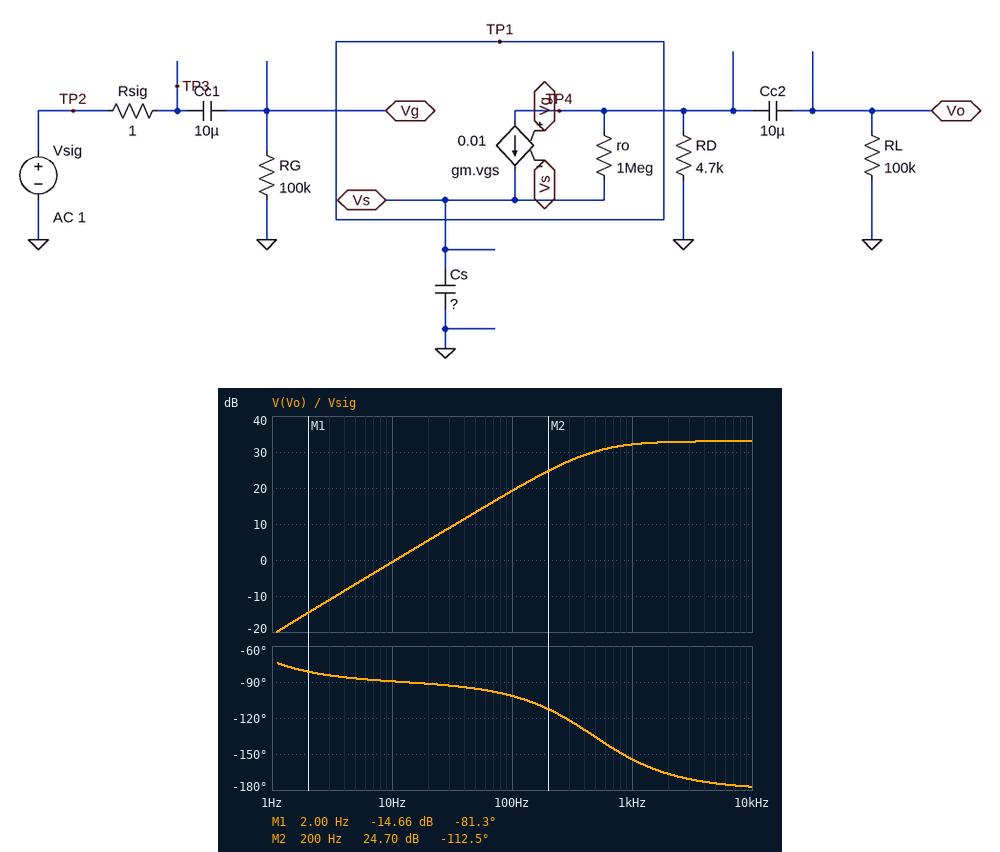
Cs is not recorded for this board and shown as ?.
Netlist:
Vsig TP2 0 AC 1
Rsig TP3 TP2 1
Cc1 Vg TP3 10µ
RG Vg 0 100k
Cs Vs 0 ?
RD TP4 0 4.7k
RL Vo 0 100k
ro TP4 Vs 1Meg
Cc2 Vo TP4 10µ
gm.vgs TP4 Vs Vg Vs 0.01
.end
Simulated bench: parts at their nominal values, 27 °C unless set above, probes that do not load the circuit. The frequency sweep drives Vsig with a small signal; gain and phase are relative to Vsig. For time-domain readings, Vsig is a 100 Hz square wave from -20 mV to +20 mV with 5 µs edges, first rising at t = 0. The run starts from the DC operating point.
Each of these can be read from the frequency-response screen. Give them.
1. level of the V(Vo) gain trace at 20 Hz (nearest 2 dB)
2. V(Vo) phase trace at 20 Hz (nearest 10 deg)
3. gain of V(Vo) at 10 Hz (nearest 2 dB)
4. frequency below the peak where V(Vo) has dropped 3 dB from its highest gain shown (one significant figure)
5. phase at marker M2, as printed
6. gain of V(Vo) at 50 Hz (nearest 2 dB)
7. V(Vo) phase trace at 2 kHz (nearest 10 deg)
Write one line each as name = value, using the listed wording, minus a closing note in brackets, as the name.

level of the V(Vo) gain trace at 20 Hz = 6 dB
V(Vo) phase trace at 20 Hz = -90 deg
gain of V(Vo) at 10 Hz = 0 dB
frequency below the peak where V(Vo) has dropped 3 dB from its highest gain shown = 500 Hz
phase at marker M2, as printed = -112.5 deg
gain of V(Vo) at 50 Hz = 14 dB
V(Vo) phase trace at 2 kHz = -170 deg
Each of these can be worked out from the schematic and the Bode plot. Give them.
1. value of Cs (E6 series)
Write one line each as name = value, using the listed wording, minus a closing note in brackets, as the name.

value of Cs = 3.3 µF
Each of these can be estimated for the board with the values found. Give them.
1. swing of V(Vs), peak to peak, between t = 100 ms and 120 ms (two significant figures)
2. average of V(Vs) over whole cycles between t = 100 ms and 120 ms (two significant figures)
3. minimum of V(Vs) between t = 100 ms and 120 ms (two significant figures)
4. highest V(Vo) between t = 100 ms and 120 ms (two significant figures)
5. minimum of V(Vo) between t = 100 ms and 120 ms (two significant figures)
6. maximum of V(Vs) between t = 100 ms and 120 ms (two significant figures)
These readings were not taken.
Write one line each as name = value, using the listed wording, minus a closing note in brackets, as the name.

swing of V(Vs), peak to peak, between t = 100 ms and 120 ms = 40 mV
average of V(Vs) over whole cycles between t = 100 ms and 120 ms = 18 mV
minimum of V(Vs) between t = 100 ms and 120 ms = -2.3 mV
highest V(Vo) between t = 100 ms and 120 ms = 1.8 V
minimum of V(Vo) between t = 100 ms and 120 ms = -1.8 V
maximum of V(Vs) between t = 100 ms and 120 ms = 38 mV
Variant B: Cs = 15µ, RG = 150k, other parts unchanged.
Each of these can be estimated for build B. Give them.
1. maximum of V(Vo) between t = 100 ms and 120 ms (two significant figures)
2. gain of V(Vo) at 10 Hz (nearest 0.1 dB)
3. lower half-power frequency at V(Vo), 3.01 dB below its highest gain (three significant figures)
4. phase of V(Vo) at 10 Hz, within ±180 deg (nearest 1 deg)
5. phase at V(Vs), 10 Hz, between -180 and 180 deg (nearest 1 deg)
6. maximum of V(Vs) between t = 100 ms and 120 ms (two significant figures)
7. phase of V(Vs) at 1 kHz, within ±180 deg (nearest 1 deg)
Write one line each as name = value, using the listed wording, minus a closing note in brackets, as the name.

maximum of V(Vo) between t = 100 ms and 120 ms = 1.7 V
gain of V(Vo) at 10 Hz = 12.5 dB
lower half-power frequency at V(Vo), 3.01 dB below its highest gain = 106 Hz
phase of V(Vo) at 10 Hz, within ±180 deg = -94 deg
phase at V(Vs), 10 Hz, between -180 and 180 deg = -5 deg
maximum of V(Vs) between t = 100 ms and 120 ms = 37 mV
phase of V(Vs) at 1 kHz, within ±180 deg = -84 deg
